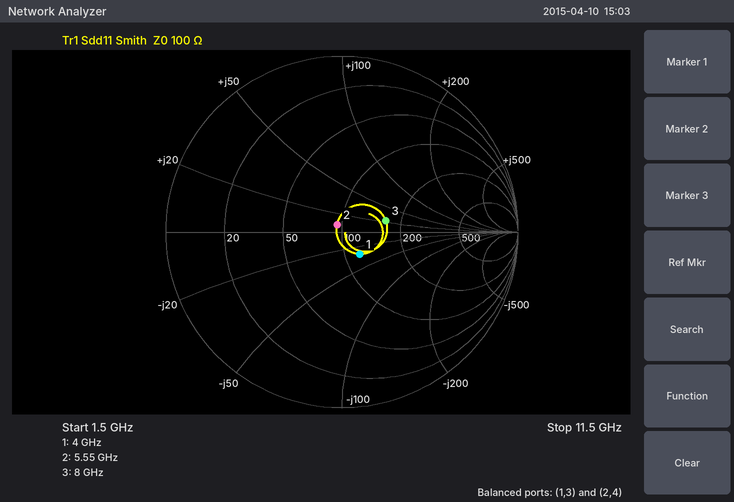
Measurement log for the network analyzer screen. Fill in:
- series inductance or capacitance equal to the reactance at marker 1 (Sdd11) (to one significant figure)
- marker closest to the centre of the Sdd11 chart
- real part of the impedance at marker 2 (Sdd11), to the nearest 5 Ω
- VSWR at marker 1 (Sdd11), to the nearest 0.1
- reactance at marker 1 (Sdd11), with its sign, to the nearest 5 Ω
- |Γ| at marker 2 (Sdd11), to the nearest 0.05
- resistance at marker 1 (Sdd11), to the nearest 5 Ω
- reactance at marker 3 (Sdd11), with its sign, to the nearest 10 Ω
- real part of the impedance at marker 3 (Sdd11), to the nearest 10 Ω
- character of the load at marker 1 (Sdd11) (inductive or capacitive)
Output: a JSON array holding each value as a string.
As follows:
["1 pF", "marker 2", "95 Ω", "1.4", "-30 Ω", "0.05", "120 Ω", "+20 Ω", "160 Ω", "capacitive"]
